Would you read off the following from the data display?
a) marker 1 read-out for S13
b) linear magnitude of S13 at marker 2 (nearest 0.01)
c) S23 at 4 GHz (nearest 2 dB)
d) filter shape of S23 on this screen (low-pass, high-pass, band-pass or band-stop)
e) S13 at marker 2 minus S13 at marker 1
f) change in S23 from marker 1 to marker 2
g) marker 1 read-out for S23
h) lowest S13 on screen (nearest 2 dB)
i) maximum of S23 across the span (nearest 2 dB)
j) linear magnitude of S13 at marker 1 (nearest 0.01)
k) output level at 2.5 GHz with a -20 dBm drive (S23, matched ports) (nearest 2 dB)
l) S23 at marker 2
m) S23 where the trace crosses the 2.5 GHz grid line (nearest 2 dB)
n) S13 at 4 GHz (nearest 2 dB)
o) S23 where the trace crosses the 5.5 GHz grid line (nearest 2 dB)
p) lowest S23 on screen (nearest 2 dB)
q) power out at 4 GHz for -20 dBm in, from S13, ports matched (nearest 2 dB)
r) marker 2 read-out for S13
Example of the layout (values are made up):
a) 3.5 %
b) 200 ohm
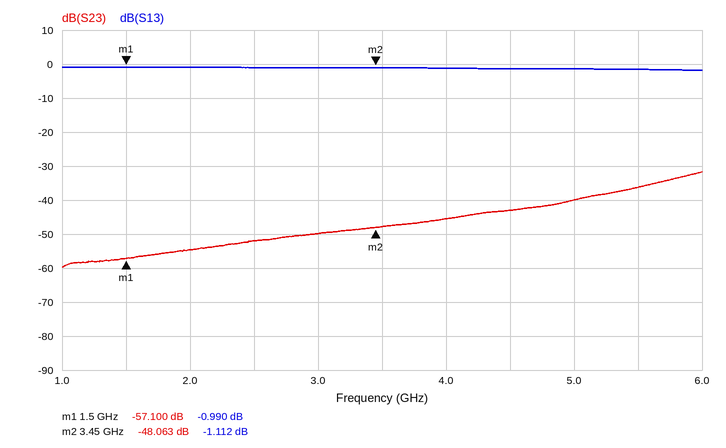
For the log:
a) -0.990 dB
b) 0.88
c) -46 dB
d) high-pass
e) -0.122 dB
f) 9.037 dB
g) -57.100 dB
h) -2 dB
i) -32 dB
j) 0.89
k) -72 dBm
l) -48.063 dB
m) -52 dB
n) -2 dB
o) -36 dB
p) -60 dB
q) -22 dBm
r) -1.112 dB
